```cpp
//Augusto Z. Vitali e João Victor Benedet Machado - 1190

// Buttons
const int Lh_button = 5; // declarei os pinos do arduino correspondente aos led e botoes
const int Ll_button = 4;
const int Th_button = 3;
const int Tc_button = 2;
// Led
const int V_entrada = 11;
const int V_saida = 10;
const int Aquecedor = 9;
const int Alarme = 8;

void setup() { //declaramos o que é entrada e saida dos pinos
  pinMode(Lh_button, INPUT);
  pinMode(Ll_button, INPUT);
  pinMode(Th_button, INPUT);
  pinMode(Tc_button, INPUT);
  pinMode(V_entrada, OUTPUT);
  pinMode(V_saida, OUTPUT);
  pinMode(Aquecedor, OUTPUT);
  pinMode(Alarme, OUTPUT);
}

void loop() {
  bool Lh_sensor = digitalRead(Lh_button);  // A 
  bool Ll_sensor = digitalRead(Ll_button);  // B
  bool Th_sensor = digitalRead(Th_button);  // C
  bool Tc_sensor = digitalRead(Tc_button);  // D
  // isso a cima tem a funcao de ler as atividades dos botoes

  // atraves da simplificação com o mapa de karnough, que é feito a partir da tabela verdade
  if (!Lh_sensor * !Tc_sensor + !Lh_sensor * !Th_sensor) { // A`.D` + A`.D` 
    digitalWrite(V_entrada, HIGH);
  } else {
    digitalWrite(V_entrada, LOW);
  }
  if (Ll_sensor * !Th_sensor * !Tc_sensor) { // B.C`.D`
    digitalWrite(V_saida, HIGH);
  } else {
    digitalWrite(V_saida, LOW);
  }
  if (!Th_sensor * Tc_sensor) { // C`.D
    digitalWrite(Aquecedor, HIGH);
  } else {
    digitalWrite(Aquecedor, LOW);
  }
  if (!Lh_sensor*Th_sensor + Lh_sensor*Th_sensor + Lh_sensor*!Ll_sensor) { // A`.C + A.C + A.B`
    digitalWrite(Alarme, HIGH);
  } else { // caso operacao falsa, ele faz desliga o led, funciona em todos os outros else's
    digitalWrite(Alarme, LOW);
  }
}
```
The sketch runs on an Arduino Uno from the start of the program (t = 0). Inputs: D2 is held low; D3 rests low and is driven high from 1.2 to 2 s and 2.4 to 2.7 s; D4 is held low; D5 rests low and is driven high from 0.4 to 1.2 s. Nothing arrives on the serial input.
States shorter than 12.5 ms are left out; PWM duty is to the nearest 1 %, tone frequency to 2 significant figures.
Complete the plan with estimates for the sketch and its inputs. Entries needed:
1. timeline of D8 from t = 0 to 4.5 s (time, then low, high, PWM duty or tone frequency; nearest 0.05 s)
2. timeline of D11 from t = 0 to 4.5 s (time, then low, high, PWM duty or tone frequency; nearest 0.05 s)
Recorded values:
0 s low; 0.4 s high; 2 s low; 2.4 s high; 2.7 s low
0 s high; 0.4 s low; 1.2 s high
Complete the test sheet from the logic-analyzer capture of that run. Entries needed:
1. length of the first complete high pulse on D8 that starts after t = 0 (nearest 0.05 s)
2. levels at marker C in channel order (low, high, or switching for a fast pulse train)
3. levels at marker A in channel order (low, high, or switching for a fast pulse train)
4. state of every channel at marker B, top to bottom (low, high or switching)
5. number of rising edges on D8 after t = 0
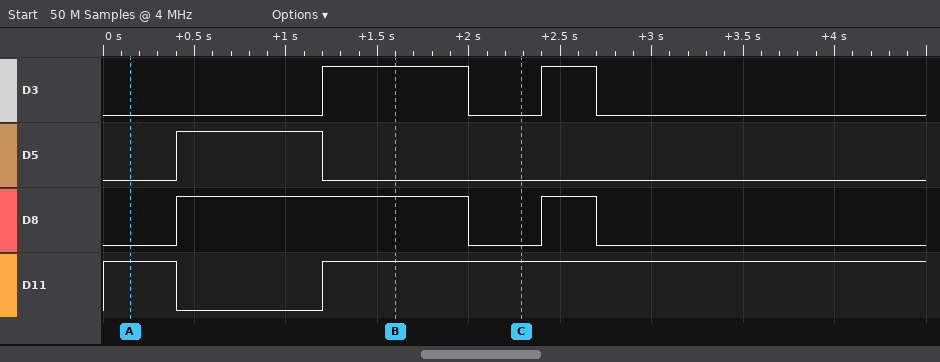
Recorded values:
1.60 s
D3 low, D5 low, D8 low, D11 high
D3 low, D5 low, D8 low, D11 high
D3 high, D5 low, D8 high, D11 high
2
